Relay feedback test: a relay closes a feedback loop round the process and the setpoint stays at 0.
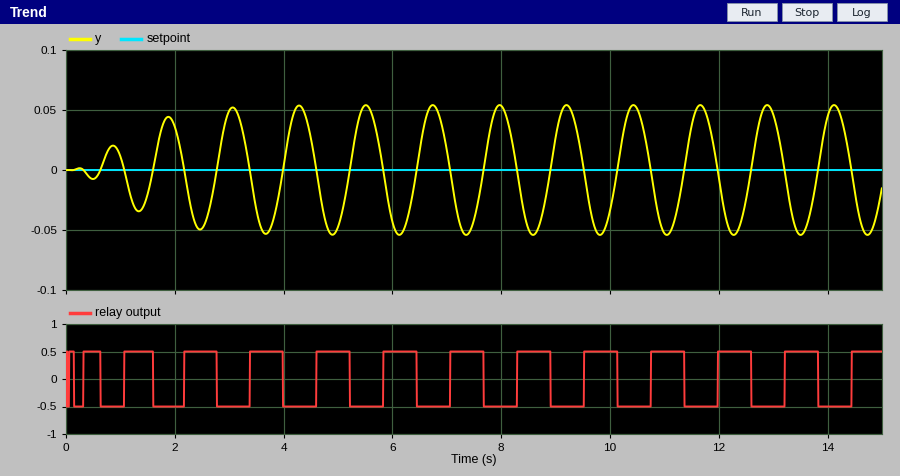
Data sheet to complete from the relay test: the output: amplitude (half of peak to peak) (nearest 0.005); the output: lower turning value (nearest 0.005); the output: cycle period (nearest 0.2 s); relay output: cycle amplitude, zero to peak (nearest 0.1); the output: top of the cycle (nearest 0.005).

0.055
-0.055
1.2 s
0.5
0.055
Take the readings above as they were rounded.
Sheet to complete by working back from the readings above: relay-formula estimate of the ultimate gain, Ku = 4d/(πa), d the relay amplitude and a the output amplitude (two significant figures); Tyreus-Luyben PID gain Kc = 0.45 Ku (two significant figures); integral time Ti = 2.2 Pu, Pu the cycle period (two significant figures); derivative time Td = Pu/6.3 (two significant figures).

12
5.4
2.6 s
0.19 s
